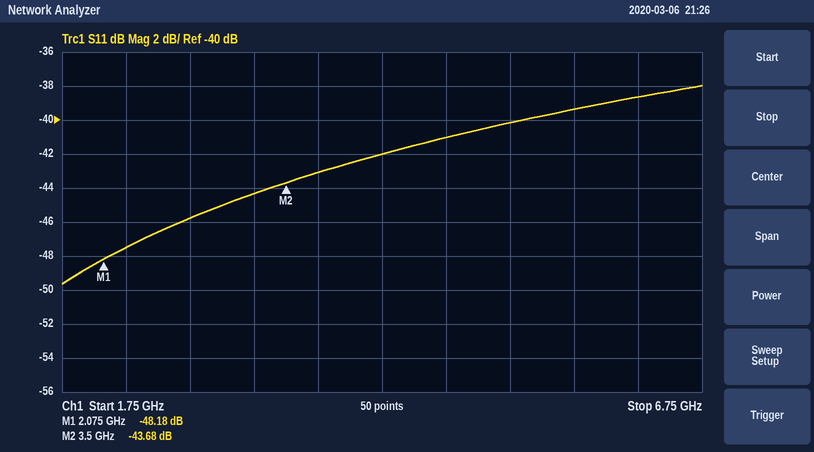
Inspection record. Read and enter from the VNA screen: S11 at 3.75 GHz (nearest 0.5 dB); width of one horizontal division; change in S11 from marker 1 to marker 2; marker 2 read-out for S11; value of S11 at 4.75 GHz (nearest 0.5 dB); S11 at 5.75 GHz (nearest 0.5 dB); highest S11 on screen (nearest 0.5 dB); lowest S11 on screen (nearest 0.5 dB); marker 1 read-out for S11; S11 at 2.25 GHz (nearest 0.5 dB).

-43.0 dB
500 MHz
4.50 dB
-43.68 dB
-41.0 dB
-39.5 dB
-38.0 dB
-49.5 dB
-48.18 dB
-47.5 dB
